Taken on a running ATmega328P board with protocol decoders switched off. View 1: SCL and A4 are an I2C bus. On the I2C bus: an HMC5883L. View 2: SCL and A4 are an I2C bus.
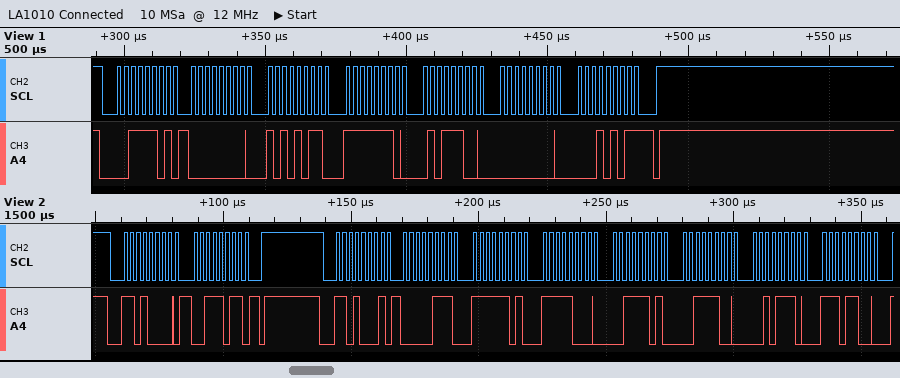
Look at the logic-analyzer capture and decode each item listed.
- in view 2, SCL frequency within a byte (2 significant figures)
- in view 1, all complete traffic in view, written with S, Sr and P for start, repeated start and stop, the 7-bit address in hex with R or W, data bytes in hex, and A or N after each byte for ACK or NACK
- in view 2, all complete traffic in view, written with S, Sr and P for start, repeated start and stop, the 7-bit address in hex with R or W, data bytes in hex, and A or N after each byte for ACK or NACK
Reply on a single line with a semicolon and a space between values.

400 kHz; S 1ER A 00 A AB A FE A 5C A 00 A 15 N P; S 68W A 3B A P S 68R A 07 A FD A F8 A 3D A 3C A 2E A EC A
